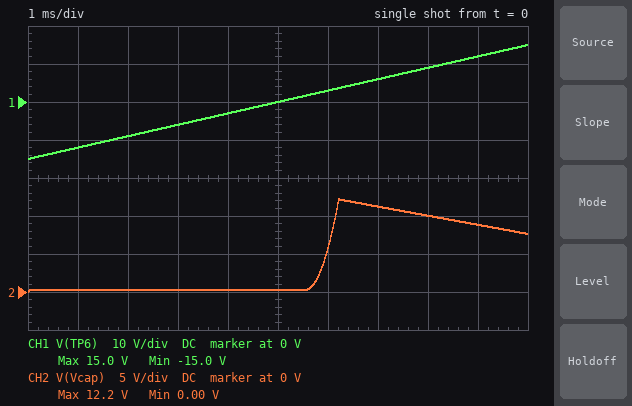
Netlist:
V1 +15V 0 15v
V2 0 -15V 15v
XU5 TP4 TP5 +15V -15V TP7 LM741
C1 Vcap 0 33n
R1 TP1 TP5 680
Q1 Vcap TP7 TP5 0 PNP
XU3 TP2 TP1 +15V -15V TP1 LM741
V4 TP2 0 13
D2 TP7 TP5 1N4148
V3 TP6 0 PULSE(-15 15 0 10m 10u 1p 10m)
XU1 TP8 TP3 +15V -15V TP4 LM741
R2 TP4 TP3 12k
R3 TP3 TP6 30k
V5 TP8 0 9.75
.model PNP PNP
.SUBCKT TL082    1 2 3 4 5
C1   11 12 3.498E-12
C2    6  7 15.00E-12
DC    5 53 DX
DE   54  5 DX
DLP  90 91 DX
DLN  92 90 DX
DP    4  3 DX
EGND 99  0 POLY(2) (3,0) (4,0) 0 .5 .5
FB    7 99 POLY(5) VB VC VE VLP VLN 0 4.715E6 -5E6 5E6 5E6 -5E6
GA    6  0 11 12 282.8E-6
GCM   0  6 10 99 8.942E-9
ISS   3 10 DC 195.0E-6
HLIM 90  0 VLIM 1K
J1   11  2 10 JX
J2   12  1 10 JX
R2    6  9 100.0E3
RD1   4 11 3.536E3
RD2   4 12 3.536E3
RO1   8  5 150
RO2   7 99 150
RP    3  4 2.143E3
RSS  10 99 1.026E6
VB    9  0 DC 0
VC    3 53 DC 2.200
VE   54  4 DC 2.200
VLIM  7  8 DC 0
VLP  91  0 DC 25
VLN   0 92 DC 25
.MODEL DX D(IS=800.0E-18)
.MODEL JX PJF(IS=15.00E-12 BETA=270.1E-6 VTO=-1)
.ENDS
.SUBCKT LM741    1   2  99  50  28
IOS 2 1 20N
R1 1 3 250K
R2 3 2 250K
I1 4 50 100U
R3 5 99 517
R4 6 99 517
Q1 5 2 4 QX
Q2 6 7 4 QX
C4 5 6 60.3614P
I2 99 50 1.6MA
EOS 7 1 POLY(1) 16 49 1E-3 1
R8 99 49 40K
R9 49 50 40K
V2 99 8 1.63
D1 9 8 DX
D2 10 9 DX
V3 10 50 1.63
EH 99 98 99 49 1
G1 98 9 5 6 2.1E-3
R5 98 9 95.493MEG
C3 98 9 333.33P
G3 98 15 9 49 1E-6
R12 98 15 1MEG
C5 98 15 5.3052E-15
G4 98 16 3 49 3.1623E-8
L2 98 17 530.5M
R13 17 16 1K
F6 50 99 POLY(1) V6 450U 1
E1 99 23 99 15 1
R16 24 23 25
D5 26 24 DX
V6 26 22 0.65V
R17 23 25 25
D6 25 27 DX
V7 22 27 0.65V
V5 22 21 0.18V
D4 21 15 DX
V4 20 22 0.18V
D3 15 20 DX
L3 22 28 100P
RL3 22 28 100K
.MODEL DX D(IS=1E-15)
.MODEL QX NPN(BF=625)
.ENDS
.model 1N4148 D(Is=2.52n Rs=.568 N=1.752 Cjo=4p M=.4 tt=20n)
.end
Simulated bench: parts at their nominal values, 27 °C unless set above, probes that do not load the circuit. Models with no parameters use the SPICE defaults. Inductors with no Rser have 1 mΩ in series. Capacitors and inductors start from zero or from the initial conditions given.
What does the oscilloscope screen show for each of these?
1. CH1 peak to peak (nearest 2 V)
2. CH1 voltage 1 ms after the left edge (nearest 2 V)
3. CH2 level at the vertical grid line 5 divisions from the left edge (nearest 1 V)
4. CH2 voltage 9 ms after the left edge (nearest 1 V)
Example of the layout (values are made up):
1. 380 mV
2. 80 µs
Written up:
1. 30 V
2. -12 V
3. 0 V
4. 9 V
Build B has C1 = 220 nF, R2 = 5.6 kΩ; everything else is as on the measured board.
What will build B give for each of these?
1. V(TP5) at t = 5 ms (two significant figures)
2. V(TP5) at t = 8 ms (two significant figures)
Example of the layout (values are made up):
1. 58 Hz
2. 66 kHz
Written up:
1. 12 V
2. 9.9 V
